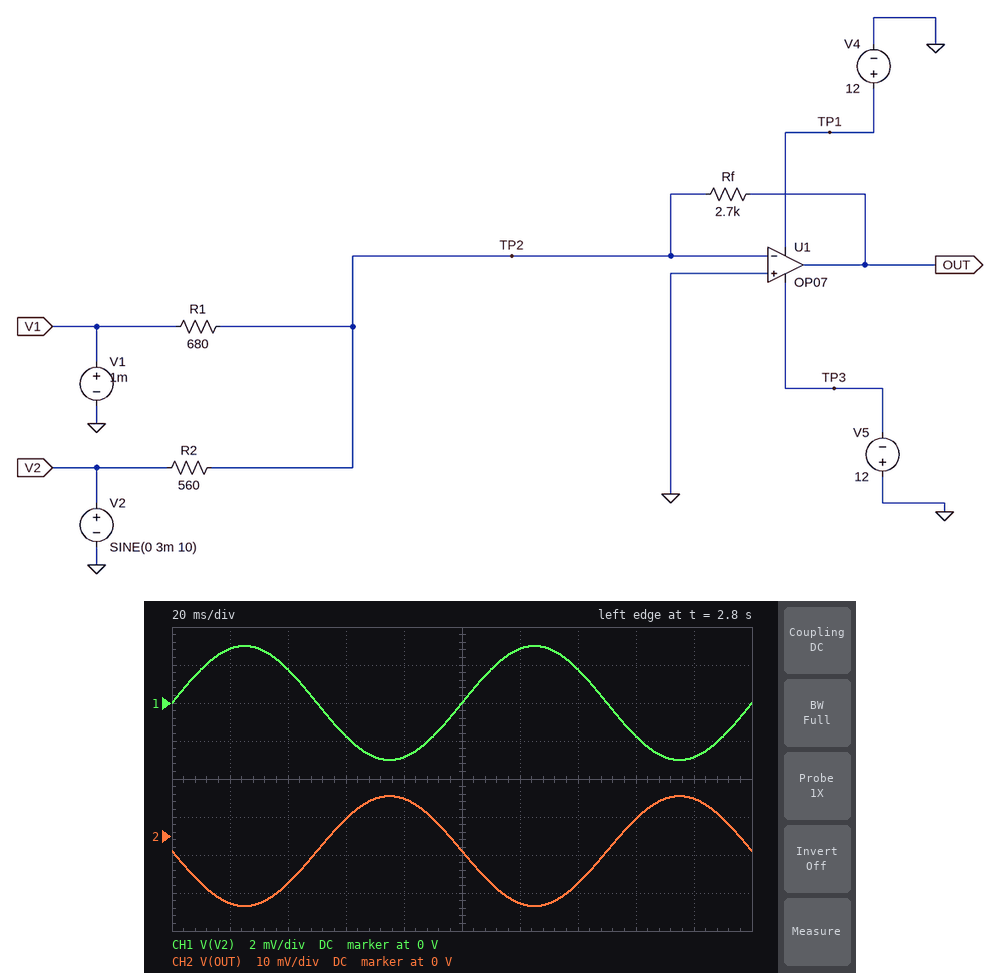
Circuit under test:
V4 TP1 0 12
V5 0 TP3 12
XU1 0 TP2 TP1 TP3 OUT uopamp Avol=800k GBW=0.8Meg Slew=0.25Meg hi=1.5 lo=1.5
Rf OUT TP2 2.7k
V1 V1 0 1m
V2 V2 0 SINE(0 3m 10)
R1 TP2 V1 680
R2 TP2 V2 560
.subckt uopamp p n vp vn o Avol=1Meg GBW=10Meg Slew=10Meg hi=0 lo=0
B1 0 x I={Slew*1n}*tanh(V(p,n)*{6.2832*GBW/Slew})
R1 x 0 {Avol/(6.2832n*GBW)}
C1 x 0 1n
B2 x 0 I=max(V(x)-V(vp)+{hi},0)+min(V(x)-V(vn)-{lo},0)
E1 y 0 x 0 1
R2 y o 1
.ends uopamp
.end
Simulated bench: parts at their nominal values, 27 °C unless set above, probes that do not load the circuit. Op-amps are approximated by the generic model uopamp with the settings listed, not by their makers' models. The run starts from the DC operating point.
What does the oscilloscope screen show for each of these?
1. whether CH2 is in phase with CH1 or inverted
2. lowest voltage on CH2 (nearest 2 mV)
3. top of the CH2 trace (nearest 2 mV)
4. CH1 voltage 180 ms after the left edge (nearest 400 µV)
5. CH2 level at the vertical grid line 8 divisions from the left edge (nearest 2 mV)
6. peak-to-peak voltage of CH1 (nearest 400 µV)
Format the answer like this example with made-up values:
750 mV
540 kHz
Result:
inverted
-18 mV
10 mV
-2.8 mV
4 mV
6.0 mV
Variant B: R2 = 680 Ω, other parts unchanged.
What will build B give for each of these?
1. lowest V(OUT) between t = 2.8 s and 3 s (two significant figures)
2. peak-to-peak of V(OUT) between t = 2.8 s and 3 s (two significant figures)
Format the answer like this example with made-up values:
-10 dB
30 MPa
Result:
-16 mV
24 mV
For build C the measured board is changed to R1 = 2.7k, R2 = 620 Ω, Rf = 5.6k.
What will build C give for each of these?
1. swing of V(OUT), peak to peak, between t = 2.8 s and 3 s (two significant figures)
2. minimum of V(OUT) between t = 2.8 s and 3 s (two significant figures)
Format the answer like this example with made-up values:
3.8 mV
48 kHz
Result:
54 mV
-29 mV
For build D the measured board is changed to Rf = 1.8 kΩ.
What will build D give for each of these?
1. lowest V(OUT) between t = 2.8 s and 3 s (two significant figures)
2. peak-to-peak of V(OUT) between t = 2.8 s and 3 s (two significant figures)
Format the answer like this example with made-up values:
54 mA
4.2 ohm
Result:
-12 mV
19 mV
